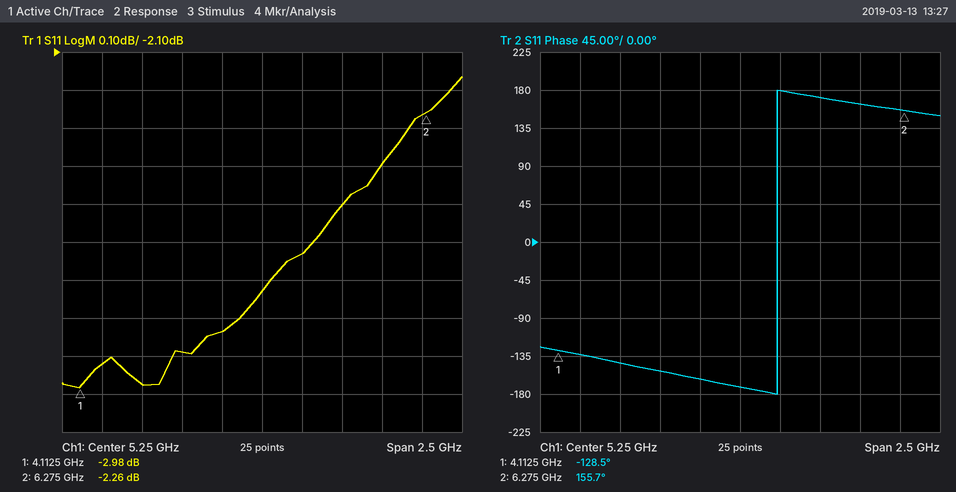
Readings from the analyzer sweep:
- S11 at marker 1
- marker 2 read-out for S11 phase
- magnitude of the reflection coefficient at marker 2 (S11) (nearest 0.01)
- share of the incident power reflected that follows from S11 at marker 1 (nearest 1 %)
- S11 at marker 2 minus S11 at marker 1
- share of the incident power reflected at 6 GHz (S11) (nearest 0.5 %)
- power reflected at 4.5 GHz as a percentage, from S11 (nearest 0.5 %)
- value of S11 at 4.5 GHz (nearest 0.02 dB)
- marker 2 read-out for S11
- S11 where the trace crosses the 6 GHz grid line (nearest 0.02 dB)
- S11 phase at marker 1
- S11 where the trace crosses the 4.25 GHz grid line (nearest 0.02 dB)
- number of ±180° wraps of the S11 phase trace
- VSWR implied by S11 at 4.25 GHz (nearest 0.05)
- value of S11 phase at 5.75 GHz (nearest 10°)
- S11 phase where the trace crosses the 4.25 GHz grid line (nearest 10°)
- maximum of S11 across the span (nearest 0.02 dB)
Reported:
-2.98 dB
155.7°
0.77
50 %
0.72 dB
57.5 %
50.5 %
-2.98 dB
-2.26 dB
-2.40 dB
-128.5°
-2.92 dB
1
6.00
170°
-130°
-2.16 dB
